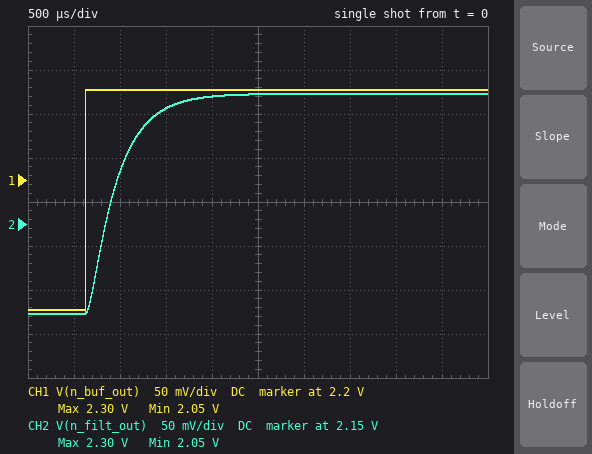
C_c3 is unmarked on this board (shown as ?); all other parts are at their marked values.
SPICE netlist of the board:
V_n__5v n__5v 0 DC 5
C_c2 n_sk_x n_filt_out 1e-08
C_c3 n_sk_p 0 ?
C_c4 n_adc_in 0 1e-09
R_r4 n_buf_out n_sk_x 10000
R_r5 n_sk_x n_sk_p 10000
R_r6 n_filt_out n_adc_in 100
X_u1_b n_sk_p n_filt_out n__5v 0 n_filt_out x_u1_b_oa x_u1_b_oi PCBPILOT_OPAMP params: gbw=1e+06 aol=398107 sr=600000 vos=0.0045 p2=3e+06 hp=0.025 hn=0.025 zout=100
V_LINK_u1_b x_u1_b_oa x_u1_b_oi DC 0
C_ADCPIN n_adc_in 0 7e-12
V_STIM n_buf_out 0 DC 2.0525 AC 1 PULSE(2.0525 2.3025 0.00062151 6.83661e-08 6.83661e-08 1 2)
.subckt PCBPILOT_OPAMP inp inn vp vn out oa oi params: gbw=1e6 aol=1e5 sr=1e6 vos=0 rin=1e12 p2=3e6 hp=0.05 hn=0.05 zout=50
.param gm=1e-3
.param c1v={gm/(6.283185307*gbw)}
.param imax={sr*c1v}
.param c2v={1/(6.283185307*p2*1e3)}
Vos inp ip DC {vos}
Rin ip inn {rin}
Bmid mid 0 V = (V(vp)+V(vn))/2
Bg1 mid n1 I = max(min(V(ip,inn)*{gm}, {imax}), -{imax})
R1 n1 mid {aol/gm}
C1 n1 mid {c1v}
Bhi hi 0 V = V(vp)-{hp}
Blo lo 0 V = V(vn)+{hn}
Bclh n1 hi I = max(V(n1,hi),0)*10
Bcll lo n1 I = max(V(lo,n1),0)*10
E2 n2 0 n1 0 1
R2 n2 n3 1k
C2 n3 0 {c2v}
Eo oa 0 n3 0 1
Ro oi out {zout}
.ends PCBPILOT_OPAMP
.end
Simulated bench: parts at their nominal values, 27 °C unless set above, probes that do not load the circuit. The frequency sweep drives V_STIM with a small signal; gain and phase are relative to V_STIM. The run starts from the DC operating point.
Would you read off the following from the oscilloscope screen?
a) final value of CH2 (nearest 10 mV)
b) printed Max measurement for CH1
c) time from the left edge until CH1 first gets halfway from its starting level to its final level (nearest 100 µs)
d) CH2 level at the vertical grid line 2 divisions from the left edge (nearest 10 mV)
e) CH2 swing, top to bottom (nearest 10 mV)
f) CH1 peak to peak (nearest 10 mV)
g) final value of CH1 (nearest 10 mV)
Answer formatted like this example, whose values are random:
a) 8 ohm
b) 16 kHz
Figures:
a) 2.30 V
b) 2.30 V
c) 600 µs
d) 2.21 V
e) 250 mV
f) 250 mV
g) 2.30 V
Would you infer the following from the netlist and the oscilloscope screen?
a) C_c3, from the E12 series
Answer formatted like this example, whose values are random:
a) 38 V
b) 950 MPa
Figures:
a) 18 nF
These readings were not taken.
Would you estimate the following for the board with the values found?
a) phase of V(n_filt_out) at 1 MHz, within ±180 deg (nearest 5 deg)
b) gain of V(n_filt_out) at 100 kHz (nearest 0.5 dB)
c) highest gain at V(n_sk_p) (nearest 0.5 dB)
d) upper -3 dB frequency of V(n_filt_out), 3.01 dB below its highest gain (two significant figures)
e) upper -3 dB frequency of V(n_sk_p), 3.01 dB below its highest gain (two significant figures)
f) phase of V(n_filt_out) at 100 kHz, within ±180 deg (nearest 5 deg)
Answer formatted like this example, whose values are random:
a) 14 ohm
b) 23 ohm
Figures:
a) 25 deg
b) -60.0 dB
c) 0 dB
d) 510 Hz
e) 510 Hz
f) 95 deg
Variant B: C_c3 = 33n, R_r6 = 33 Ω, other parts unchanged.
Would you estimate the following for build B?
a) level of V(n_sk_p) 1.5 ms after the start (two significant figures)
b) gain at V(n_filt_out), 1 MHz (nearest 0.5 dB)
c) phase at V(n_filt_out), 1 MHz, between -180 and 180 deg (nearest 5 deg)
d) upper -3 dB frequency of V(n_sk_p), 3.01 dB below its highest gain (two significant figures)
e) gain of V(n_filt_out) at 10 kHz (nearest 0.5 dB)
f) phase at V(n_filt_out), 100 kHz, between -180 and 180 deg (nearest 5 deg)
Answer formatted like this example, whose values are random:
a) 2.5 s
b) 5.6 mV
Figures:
a) 2.2 V
b) -39.0 dB
c) 20 deg
d) 260 Hz
e) -42.5 dB
f) 90 deg
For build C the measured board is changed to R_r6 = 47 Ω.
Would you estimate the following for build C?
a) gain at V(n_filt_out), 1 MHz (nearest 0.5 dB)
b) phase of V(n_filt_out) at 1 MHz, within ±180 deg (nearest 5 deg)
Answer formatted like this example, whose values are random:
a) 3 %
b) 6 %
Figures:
a) -39.5 dB
b) 20 deg
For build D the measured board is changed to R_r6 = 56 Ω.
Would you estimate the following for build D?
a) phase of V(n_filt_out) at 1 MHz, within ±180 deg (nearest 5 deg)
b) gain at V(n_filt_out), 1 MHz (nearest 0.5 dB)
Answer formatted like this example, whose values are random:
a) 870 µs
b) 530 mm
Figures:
a) 20 deg
b) -40.0 dB
